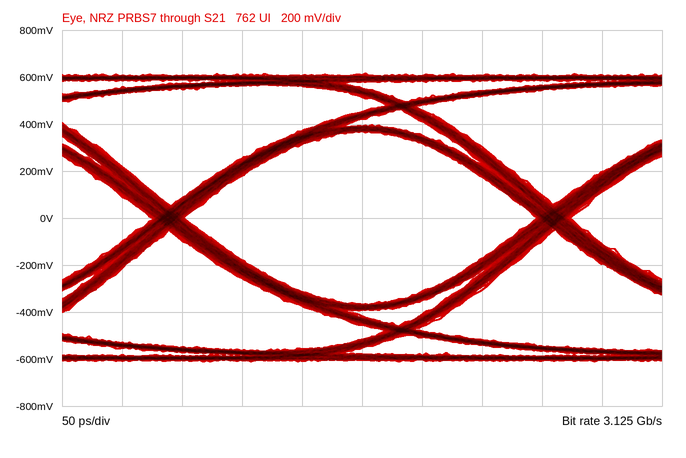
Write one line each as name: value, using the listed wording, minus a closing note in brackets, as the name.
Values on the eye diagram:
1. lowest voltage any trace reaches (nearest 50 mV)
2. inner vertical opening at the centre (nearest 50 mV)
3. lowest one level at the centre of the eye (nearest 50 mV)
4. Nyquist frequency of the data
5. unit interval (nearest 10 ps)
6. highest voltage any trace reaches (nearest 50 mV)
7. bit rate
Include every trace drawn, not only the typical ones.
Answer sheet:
lowest voltage any trace reaches: -600 mV
inner vertical opening at the centre: 750 mV
lowest one level at the centre of the eye: 350 mV
Nyquist frequency of the data: 1.5625 GHz
unit interval: 320 ps
highest voltage any trace reaches: 600 mV
bit rate: 3.125 Gb/s
